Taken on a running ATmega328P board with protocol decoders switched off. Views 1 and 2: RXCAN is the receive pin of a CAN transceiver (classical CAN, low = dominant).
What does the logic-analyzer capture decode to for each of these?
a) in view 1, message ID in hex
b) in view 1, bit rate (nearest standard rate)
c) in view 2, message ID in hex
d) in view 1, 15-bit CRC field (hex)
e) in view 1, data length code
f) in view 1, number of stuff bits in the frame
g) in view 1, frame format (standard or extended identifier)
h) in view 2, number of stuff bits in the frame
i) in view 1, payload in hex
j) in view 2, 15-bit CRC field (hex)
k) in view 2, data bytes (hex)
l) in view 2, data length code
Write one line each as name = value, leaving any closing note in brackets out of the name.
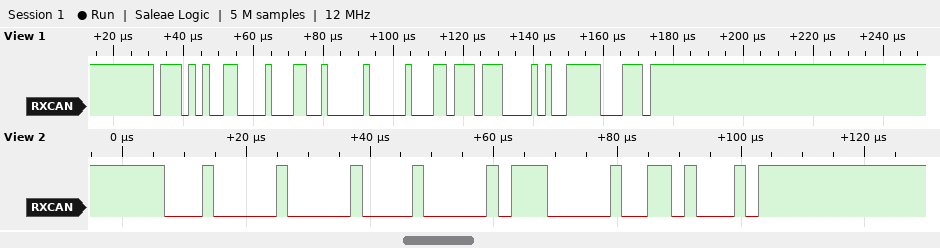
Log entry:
in view 1, message ID in hex = 0x753
in view 1, bit rate = 500 kbit/s
in view 2, message ID in hex = 0x100
in view 1, 15-bit CRC field = 0x29F3
in view 1, data length code = 4
in view 1, number of stuff bits in the frame = 3
in view 1, frame format = standard
in view 2, number of stuff bits in the frame = 4
in view 1, payload in hex = 64 00 1B B8
in view 2, 15-bit CRC field = 0x4068
in view 2, data bytes = 03
in view 2, data length code = 1
